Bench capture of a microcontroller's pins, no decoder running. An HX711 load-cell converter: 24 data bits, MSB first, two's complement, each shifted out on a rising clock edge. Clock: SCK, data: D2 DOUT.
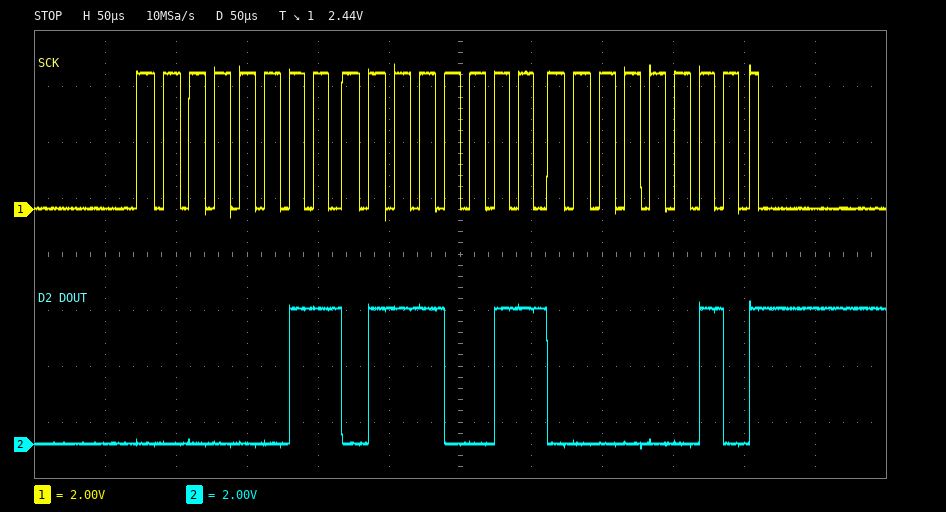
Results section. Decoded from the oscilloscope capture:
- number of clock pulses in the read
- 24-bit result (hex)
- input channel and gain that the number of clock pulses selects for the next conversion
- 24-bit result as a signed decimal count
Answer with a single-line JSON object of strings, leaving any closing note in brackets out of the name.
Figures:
{"number of clock pulses in the read": "25", "24-bit result": "0x037302", "input channel and gain that the number of clock pulses selects for the next conversion": "channel A, gain 128", "24-bit result as a signed decimal count": "226050"}
